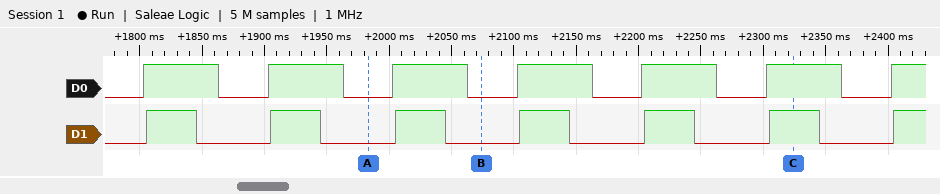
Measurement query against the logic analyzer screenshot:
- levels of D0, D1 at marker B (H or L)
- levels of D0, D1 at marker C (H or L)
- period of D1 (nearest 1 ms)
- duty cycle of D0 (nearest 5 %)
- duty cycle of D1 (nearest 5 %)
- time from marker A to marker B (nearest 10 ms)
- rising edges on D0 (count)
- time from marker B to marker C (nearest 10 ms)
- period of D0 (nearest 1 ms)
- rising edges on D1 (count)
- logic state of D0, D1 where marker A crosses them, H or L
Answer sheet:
D0=L, D1=L
D0=H, D1=H
100 ms
60 %
40 %
90 ms
7
250 ms
100 ms
7
D0=L, D1=L
